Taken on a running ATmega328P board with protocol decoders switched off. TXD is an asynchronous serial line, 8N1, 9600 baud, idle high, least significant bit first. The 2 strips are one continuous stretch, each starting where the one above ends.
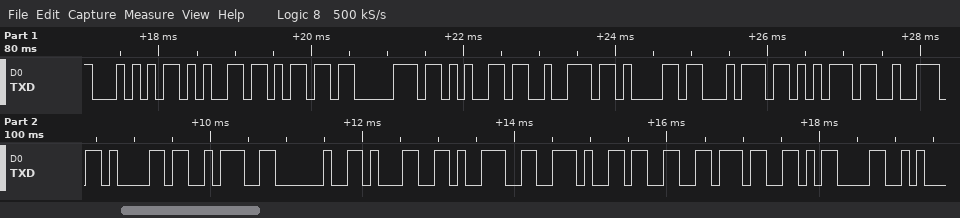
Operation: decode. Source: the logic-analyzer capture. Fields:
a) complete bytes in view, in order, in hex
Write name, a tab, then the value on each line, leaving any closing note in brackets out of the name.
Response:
complete bytes in view, in order, in hex	0x54 0x65 0x6D 0x70 0x65 0x72 0x61 0x74 0x75 0x72 0x61 0x3A 0x20 0x31 0x39 0x2E 0x33 0x37 0x0D
